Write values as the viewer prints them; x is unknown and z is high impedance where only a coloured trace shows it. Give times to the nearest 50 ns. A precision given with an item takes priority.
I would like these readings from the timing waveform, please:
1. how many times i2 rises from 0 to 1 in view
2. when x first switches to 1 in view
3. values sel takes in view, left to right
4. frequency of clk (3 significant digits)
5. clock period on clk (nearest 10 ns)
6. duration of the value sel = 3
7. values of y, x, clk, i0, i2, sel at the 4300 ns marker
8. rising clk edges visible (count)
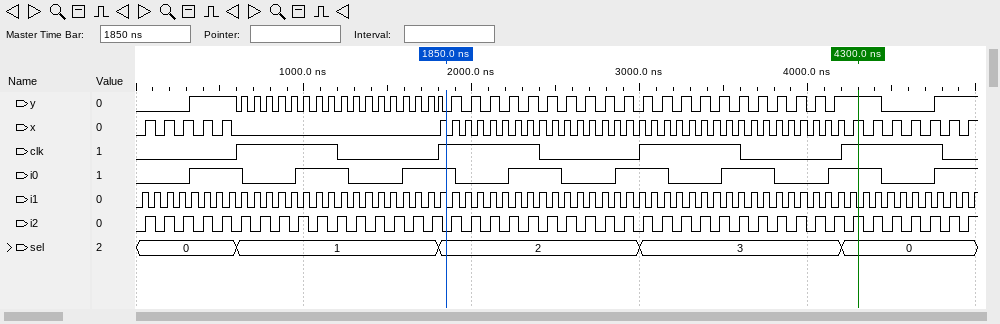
44
50 ns
0, 1, 2, 3, 0
833 kHz
1200 ns
1200 ns
y=1, x=1, clk=1, i0=1, i2=1, sel=0
4
